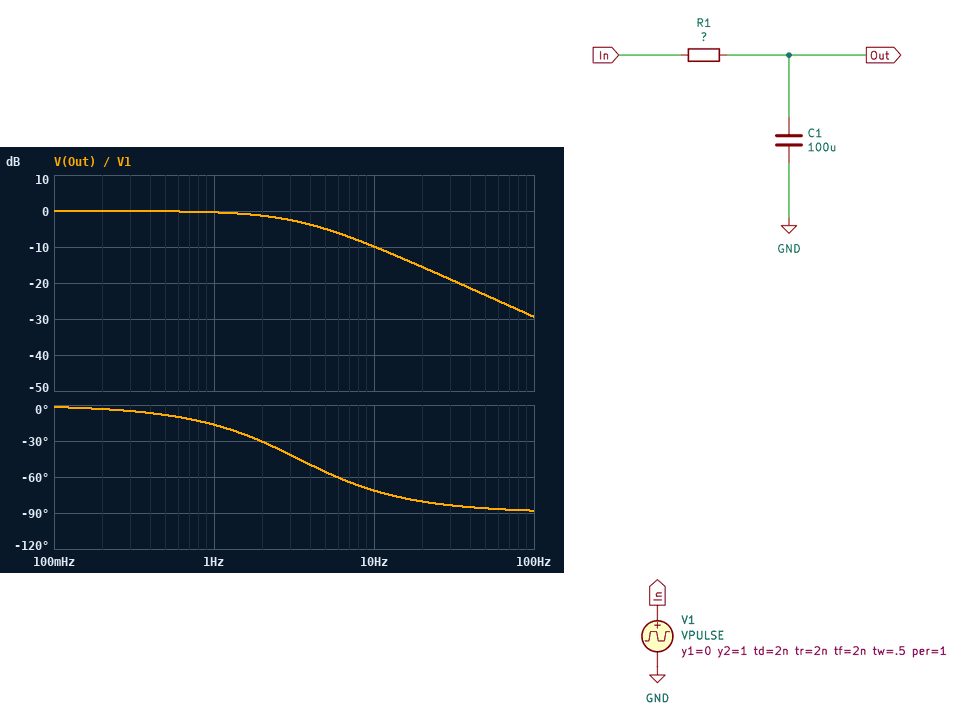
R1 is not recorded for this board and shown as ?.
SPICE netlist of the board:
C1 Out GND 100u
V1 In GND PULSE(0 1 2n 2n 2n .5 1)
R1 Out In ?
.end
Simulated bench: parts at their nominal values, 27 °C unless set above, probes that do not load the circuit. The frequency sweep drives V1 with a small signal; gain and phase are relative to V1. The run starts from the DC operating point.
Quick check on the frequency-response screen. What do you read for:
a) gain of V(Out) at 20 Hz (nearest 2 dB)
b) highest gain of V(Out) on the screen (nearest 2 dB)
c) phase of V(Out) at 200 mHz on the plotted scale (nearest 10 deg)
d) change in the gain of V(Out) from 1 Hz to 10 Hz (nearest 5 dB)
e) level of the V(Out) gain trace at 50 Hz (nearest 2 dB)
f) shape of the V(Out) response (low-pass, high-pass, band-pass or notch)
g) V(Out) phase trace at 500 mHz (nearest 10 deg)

-16 dB
0 dB
0 deg
-10 dB
-24 dB
low-pass
-10 deg
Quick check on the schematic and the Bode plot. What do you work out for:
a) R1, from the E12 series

470 Ω
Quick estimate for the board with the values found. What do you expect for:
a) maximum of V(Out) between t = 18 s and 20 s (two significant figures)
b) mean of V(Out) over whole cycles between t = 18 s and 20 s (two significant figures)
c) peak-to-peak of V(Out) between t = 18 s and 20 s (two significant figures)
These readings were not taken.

1.0 V
500 mV
1.0 V
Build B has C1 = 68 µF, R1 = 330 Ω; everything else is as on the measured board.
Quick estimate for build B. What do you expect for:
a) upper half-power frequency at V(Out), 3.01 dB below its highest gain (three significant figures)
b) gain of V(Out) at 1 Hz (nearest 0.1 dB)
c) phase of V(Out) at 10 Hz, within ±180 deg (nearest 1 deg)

7.09 Hz
-0.1 dB
-55 deg
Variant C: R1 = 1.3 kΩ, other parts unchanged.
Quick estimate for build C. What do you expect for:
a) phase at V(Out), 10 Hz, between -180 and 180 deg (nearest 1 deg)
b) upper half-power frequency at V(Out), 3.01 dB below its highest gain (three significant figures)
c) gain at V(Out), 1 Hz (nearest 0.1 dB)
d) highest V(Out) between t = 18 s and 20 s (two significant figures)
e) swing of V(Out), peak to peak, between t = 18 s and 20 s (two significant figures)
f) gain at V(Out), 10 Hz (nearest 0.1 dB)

-83 deg
1.22 Hz
-2.2 dB
980 mV
960 mV
-18.3 dB
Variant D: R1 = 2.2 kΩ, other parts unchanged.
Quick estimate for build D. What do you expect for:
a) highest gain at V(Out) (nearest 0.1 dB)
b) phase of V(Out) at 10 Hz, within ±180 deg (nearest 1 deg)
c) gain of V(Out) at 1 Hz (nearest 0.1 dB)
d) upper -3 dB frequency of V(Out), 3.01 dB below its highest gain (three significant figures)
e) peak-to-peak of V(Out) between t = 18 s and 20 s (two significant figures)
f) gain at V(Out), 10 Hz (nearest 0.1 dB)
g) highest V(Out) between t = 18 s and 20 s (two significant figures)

0 dB
-86 deg
-4.6 dB
723 mHz
810 mV
-22.8 dB
910 mV
